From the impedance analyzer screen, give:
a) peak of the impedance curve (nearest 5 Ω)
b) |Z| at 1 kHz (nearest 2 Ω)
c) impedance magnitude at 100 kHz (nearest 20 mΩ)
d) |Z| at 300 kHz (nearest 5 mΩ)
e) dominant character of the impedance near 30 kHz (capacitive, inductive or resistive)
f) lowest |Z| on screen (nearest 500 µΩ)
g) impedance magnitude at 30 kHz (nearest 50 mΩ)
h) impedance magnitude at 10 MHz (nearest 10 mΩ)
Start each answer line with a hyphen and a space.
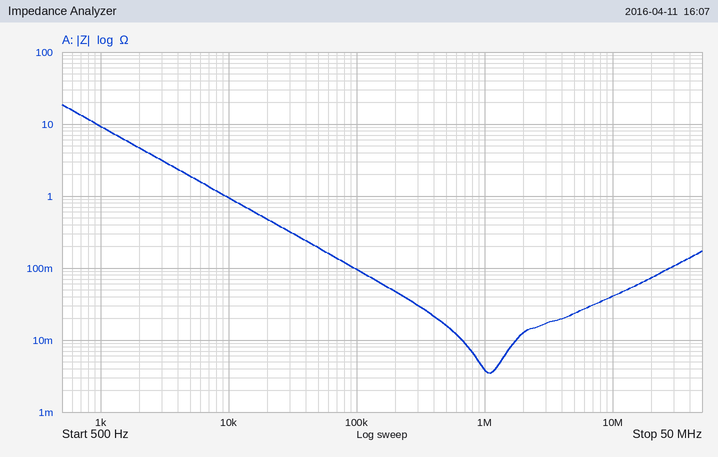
- 20 Ω
- 10 Ω
- 100 mΩ
- 30 mΩ
- capacitive
- 3.5 mΩ
- 300 mΩ
- 40 mΩ
